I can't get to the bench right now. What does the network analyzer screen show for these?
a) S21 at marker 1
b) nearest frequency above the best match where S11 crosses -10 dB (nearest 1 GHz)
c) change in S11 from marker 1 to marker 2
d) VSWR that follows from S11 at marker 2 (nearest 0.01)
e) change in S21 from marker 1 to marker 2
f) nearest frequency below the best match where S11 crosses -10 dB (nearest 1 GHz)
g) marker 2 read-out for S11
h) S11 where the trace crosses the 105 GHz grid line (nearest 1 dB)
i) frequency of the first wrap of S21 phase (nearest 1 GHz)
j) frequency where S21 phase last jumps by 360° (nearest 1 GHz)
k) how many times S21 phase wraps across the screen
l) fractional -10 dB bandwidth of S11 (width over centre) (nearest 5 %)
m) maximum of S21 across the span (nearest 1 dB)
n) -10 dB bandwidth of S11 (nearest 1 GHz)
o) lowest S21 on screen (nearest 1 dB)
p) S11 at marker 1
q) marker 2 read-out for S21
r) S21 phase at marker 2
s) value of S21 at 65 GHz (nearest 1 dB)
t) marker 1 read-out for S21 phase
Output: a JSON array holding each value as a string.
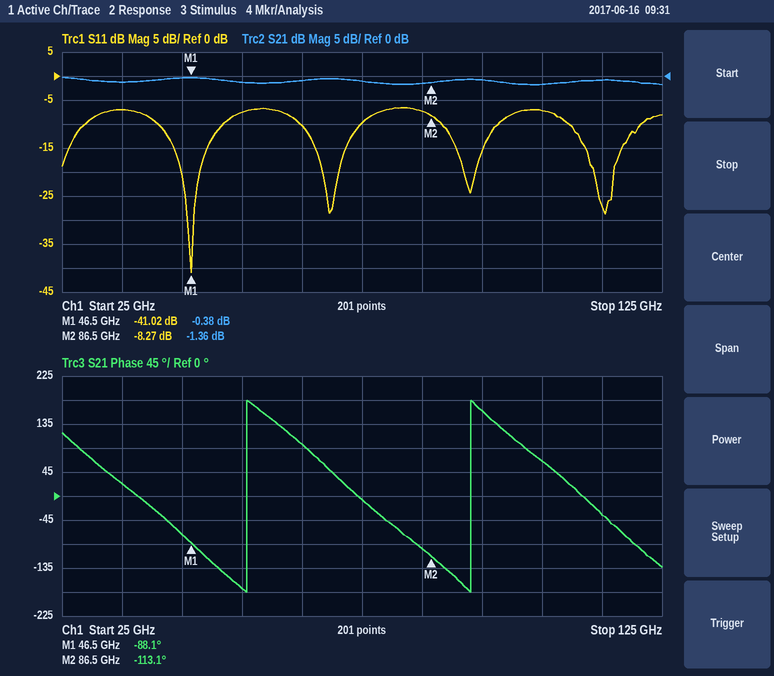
["-0.38 dB", "52 GHz", "32.75 dB", "2.26", "-0.98 dB", "41 GHz", "-8.27 dB", "-7 dB", "56 GHz", "93 GHz", "2", "25 %", "0 dB", "11 GHz", "-2 dB", "-41.02 dB", "-1.36 dB", "-113.1°", "-1 dB", "-88.1°"]
